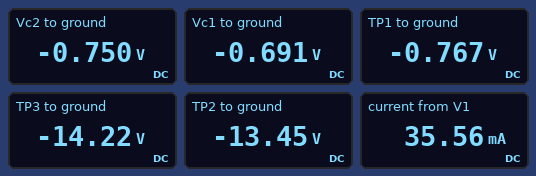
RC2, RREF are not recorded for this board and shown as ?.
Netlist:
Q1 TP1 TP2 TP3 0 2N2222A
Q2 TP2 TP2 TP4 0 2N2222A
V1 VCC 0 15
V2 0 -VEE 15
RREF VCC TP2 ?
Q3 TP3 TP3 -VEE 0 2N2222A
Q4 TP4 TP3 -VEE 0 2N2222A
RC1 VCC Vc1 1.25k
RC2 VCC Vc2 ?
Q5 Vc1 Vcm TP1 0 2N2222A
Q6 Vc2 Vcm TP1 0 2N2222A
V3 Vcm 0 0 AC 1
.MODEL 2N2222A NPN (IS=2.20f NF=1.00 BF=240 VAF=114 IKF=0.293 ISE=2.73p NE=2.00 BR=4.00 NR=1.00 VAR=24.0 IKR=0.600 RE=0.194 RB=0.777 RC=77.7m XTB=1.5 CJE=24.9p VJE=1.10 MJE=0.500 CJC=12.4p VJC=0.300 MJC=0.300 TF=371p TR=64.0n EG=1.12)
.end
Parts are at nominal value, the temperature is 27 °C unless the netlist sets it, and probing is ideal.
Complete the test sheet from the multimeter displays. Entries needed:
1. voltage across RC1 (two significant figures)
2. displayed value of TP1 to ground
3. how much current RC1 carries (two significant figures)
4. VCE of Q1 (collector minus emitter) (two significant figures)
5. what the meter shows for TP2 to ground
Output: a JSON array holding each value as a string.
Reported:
["16 V", "-0.767 V", "13 mA", "13 V", "-13.45 V"]
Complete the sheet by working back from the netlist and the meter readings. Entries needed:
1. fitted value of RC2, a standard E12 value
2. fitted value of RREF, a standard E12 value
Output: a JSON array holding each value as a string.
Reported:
["3.9 kΩ", "1.5 kΩ"]
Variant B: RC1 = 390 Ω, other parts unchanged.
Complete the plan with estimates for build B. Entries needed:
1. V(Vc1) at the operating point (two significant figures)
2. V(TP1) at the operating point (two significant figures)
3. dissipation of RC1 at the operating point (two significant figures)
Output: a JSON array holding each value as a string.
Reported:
["9.9 V", "-760 mV", "67 mW"]
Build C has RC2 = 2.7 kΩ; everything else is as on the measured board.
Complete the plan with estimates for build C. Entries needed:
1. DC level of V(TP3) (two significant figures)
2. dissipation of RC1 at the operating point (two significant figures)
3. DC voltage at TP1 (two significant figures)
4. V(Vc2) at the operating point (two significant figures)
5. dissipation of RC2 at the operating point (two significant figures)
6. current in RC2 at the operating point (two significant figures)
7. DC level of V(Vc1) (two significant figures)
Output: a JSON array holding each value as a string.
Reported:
["-14 V", "170 mW", "-760 mV", "-740 mV", "92 mW", "5.8 mA", "250 mV"]
